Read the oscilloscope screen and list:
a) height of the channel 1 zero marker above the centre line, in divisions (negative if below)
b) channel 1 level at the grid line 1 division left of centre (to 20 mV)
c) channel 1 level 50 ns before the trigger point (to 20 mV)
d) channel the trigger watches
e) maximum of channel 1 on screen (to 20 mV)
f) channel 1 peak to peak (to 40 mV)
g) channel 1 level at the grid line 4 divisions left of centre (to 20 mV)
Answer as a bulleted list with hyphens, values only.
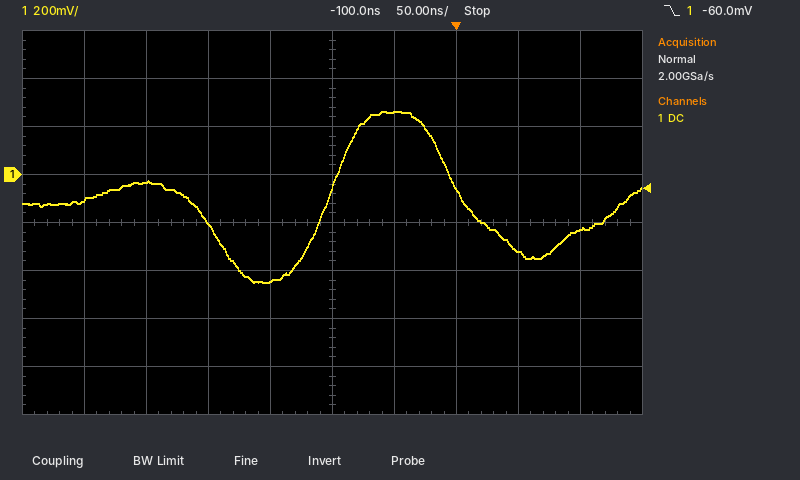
- +1.0 div
- -440 mV
- 260 mV
- channel 1
- 260 mV
- 720 mV
- -100 mV
